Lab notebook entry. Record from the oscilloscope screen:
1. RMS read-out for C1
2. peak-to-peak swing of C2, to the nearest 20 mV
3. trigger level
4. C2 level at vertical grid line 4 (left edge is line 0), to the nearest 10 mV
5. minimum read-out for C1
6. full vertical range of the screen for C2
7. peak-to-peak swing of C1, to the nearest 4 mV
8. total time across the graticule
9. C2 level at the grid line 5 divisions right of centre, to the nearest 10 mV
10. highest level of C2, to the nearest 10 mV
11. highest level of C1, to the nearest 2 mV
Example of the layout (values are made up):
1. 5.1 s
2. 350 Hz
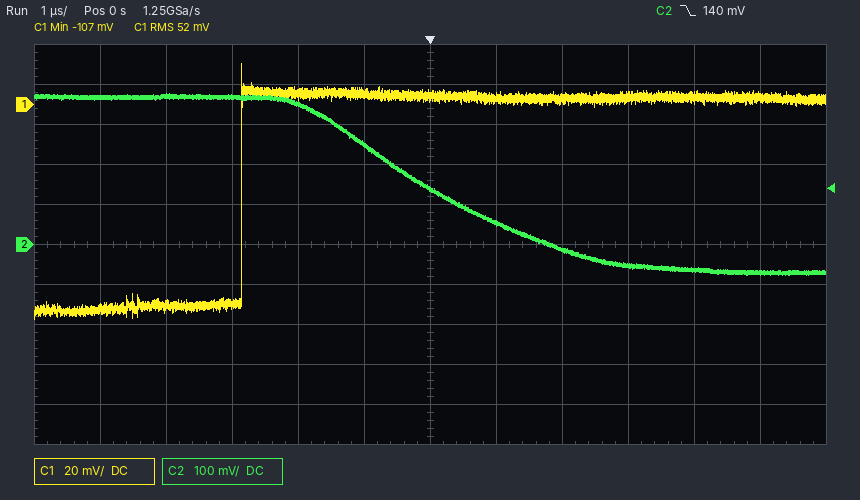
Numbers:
1. 52 mV
2. 460 mV
3. 140 mV
4. 350 mV
5. -107 mV
6. 1 V
7. 128 mV
8. 12 µs
9. -70 mV
10. 380 mV
11. 20 mV
